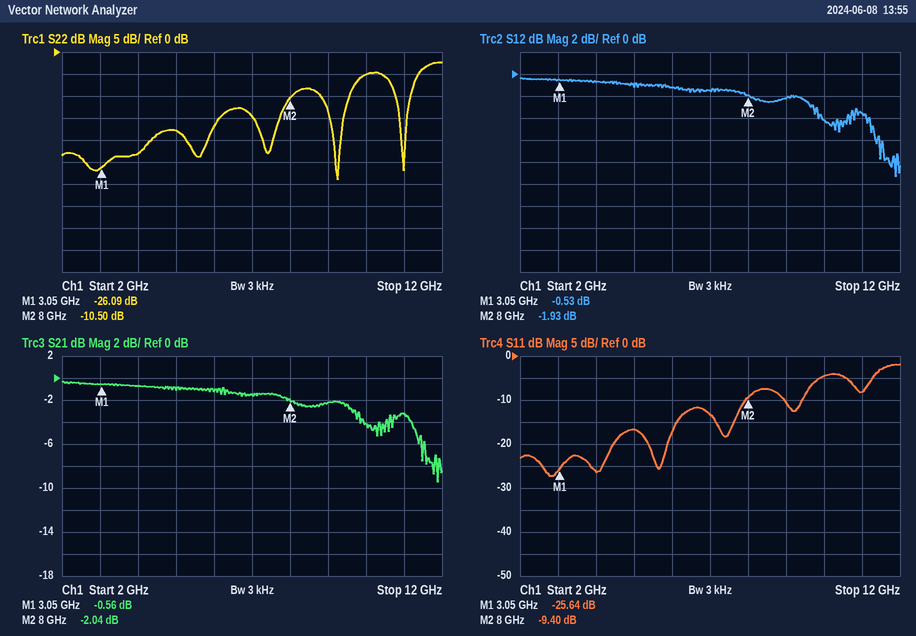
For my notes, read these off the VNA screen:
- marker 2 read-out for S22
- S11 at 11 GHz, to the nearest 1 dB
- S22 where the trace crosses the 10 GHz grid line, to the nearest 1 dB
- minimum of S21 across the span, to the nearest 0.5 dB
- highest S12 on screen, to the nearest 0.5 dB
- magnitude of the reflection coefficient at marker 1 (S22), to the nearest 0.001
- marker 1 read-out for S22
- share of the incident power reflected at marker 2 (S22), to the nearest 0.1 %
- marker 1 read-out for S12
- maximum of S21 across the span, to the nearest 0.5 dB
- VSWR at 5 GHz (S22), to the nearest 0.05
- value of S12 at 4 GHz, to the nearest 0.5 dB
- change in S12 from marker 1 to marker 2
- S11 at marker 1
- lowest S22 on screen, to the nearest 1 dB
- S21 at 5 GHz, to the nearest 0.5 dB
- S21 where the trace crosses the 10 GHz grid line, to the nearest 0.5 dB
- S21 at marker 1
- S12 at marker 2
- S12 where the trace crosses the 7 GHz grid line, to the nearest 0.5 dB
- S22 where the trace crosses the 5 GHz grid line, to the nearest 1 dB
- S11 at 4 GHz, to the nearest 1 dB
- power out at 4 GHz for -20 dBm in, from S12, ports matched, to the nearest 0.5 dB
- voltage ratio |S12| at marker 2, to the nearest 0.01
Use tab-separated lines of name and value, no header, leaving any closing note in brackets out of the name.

marker 2 read-out for S22	-10.50 dB
S11 at 11 GHz, to the nearest 1 dB	-8 dB
S22 where the trace crosses the 10 GHz grid line, to the nearest 1 dB	-5 dB
minimum of S21 across the span, to the nearest 0.5 dB	-9.5 dB
highest S12 on screen, to the nearest 0.5 dB	-0.5 dB
magnitude of the reflection coefficient at marker 1 (S22), to the nearest 0.001	0.050
marker 1 read-out for S22	-26.09 dB
share of the incident power reflected at marker 2 (S22), to the nearest 0.1 %	8.9 %
marker 1 read-out for S12	-0.53 dB
maximum of S21 across the span, to the nearest 0.5 dB	-0.5 dB
VSWR at 5 GHz (S22), to the nearest 0.05	1.30
value of S12 at 4 GHz, to the nearest 0.5 dB	-0.5 dB
change in S12 from marker 1 to marker 2	-1.40 dB
S11 at marker 1	-25.64 dB
lowest S22 on screen, to the nearest 1 dB	-29 dB
S21 at 5 GHz, to the nearest 0.5 dB	-1.0 dB
S21 where the trace crosses the 10 GHz grid line, to the nearest 0.5 dB	-4.0 dB
S21 at marker 1	-0.56 dB
S12 at marker 2	-1.93 dB
S12 where the trace crosses the 7 GHz grid line, to the nearest 0.5 dB	-1.5 dB
S22 where the trace crosses the 5 GHz grid line, to the nearest 1 dB	-18 dB
S11 at 4 GHz, to the nearest 1 dB	-26 dB
power out at 4 GHz for -20 dBm in, from S12, ports matched, to the nearest 0.5 dB	-20.5 dBm
voltage ratio |S12| at marker 2, to the nearest 0.01	0.80
